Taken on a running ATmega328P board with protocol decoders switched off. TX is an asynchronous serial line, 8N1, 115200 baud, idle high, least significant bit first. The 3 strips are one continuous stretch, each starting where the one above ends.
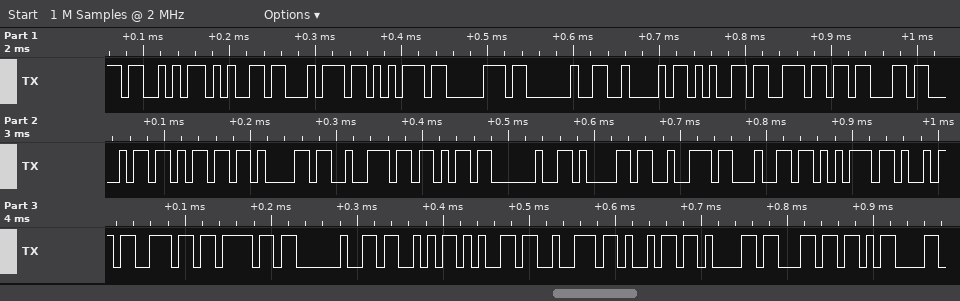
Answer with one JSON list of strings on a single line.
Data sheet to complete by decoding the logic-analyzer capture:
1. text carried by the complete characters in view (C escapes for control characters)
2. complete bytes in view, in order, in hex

["\"Setup Benchmark arduino Serial\\r\"", "53 65 74 75 70 20 42 65 6E 63 68 6D 61 72 6B 20 61 72 64 75 69 6E 6F 20 53 65 72 69 61 6C 0D"]
